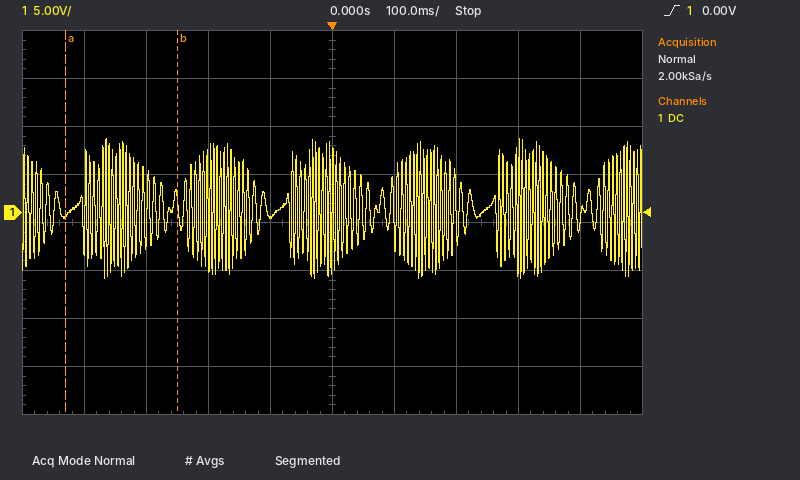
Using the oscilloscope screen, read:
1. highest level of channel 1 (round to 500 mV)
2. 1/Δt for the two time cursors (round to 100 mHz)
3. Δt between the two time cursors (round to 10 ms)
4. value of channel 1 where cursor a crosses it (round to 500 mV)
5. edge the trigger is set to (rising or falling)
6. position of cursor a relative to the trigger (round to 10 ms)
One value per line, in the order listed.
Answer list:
8.0 V
5.6 Hz
180 ms
-500 mV
rising
-430 ms
